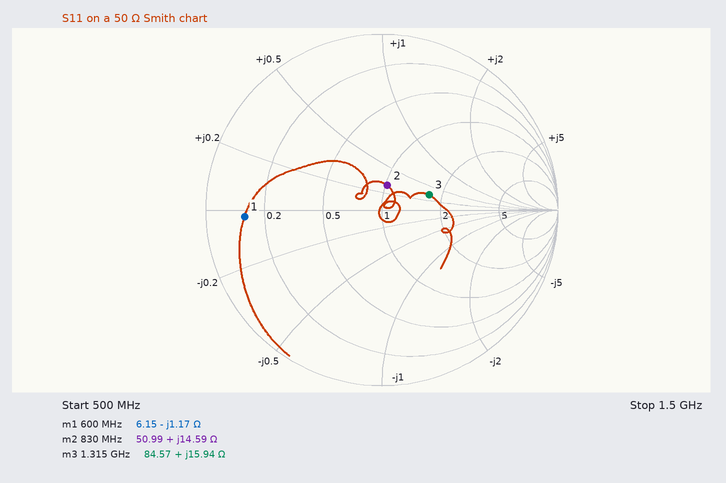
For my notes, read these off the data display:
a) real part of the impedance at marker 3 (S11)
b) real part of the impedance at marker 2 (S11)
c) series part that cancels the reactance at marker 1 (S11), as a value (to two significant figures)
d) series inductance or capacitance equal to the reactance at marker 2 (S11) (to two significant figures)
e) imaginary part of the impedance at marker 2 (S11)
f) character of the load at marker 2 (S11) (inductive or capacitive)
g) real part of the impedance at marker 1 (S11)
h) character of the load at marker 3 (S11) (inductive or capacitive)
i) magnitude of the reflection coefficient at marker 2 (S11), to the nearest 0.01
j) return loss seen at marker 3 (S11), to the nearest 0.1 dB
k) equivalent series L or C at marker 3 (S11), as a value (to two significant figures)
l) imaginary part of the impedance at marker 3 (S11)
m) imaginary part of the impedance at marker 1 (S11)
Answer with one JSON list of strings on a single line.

["84.57 Ω", "50.99 Ω", "310 pH", "2.8 nH", "+14.59 Ω", "inductive", "6.15 Ω", "inductive", "0.14", "11.0 dB", "1.9 nH", "+15.94 Ω", "-1.17 Ω"]
